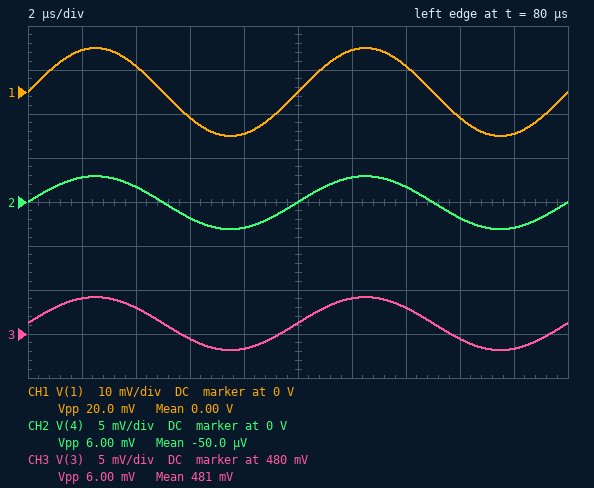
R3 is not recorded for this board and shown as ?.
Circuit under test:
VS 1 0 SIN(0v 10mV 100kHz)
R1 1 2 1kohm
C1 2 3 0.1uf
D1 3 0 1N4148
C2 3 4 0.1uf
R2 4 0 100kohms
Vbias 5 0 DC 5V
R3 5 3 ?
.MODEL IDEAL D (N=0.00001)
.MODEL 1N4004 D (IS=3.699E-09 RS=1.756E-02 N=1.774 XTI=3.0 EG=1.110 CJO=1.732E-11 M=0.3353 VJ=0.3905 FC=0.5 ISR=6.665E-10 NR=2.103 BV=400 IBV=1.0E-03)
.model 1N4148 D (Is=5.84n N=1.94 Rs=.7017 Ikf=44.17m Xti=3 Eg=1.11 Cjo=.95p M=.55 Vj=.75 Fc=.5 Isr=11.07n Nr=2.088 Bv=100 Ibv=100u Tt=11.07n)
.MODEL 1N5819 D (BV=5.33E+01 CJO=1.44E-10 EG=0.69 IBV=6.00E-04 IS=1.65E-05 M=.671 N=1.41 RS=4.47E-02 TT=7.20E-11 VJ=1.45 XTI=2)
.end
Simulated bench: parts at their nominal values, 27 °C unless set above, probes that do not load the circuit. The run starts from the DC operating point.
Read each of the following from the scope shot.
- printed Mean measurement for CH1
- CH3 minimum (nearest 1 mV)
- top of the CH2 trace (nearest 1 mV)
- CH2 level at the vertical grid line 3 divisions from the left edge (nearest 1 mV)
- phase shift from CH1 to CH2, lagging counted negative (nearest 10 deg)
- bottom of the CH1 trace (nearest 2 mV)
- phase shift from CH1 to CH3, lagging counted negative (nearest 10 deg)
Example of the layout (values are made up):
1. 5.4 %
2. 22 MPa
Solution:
1. 0.00 V
2. 478 mV
3. 3 mV
4. -2 mV
5. 0 deg
6. -10 mV
7. 0 deg
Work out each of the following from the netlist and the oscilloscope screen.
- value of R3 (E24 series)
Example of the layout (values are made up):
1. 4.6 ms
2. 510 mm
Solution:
1. 36 kΩ
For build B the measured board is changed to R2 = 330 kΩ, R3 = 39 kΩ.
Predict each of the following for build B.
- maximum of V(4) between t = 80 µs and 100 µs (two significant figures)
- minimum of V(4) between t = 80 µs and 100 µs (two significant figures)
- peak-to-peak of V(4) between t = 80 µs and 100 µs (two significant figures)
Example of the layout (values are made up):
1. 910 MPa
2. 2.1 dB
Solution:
1. 3.1 mV
2. -3.3 mV
3. 6.4 mV
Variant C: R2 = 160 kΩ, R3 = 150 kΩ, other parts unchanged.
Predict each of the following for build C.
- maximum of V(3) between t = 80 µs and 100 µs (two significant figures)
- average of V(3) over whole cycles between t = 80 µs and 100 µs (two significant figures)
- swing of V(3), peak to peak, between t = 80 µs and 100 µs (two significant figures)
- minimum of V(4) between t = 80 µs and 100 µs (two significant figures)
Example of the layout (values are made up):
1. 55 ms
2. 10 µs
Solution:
1. 410 mV
2. 400 mV
3. 13 mV
4. -6.5 mV
